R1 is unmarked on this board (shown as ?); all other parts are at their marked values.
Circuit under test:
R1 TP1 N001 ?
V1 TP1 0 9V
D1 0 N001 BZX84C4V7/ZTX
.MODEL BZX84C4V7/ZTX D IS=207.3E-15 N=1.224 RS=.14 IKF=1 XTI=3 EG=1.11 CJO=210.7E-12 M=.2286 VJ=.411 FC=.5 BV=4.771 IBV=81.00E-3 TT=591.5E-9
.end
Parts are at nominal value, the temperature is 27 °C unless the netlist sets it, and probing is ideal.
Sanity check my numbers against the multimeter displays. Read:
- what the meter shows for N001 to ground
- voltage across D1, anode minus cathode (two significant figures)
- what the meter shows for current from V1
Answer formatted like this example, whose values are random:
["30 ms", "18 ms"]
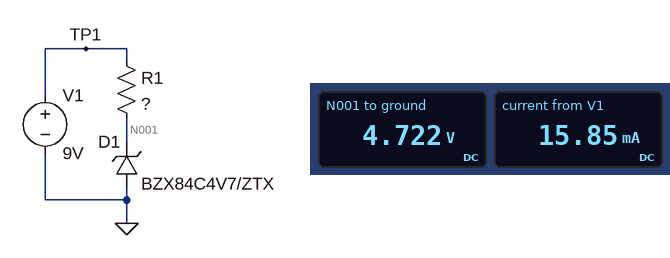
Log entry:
["4.722 V", "-4.7 V", "15.85 mA"]
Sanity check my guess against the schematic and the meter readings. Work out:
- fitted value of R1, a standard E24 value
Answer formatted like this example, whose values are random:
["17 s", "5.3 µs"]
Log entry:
["270 Ω"]
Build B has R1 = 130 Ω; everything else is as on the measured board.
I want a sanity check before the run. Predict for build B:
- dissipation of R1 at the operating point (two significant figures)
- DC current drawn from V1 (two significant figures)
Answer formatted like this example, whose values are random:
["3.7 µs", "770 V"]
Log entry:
["140 mW", "33 mA"]
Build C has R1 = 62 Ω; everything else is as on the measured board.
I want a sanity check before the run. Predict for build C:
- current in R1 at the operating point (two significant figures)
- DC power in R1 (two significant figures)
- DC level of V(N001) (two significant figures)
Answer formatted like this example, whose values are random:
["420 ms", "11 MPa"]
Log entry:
["68 mA", "290 mW", "4.8 V"]
